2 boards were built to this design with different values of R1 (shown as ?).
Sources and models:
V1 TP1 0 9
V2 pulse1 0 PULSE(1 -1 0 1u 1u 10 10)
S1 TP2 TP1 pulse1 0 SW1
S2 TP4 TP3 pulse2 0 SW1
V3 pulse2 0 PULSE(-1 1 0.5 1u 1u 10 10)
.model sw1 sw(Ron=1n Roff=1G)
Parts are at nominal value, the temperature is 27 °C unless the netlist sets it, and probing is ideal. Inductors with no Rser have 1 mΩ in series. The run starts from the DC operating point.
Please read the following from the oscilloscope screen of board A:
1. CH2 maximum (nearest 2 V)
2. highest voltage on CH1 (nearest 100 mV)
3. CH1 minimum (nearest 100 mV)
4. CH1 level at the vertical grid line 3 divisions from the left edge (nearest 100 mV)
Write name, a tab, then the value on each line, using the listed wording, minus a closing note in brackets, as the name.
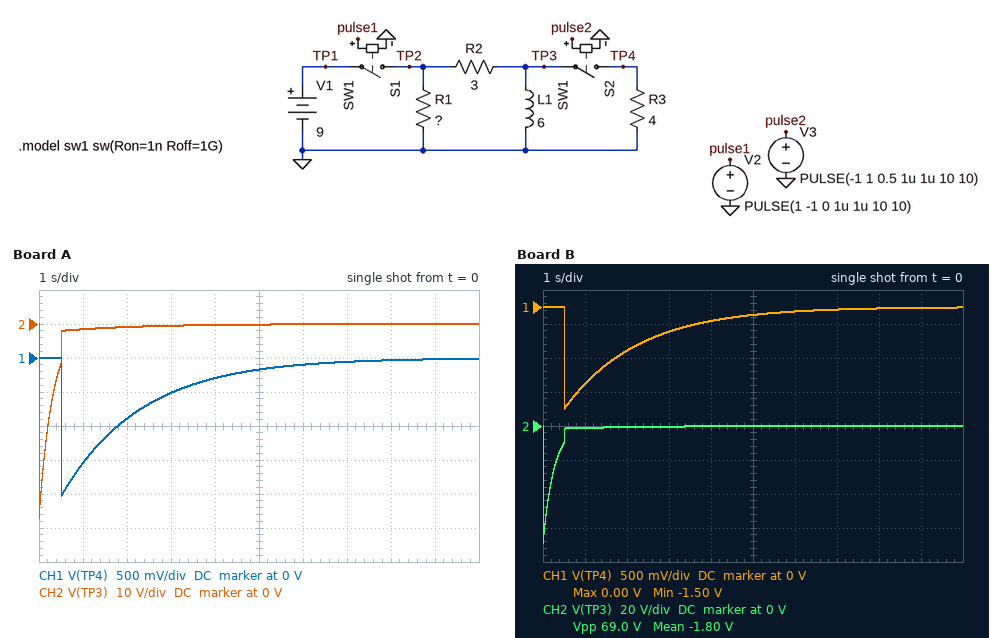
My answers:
CH2 maximum	0 V
highest voltage on CH1	0 V
CH1 minimum	-2.0 V
CH1 level at the vertical grid line 3 divisions from the left edge	-500 mV
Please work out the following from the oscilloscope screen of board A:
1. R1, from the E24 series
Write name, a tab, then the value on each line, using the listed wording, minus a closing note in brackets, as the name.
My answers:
R1, from the E24 series	16 Ω
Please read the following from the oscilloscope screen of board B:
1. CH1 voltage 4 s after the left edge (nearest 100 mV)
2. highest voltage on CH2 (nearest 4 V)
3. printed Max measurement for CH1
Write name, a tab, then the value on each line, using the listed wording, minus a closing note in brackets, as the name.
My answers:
CH1 voltage 4 s after the left edge	-200 mV
highest voltage on CH2	0 V
printed Max measurement for CH1	0.00 V
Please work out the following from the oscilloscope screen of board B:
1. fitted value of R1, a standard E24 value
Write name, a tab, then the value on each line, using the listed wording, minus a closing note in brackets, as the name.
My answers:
fitted value of R1, a standard E24 value	20 Ω
